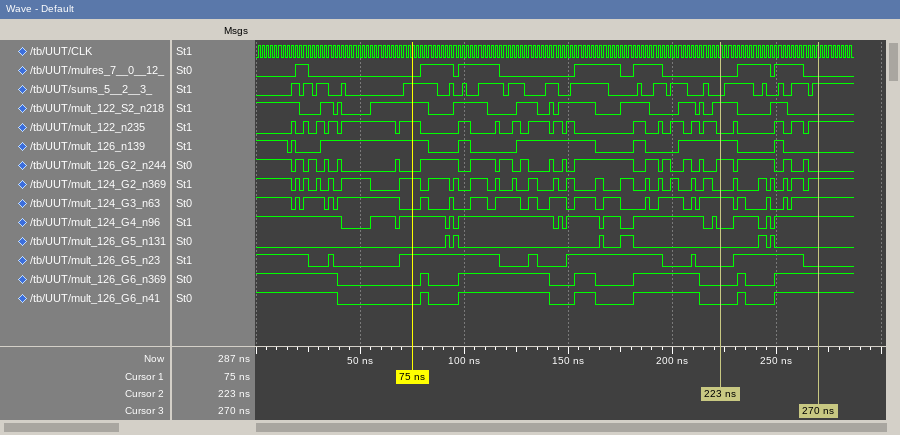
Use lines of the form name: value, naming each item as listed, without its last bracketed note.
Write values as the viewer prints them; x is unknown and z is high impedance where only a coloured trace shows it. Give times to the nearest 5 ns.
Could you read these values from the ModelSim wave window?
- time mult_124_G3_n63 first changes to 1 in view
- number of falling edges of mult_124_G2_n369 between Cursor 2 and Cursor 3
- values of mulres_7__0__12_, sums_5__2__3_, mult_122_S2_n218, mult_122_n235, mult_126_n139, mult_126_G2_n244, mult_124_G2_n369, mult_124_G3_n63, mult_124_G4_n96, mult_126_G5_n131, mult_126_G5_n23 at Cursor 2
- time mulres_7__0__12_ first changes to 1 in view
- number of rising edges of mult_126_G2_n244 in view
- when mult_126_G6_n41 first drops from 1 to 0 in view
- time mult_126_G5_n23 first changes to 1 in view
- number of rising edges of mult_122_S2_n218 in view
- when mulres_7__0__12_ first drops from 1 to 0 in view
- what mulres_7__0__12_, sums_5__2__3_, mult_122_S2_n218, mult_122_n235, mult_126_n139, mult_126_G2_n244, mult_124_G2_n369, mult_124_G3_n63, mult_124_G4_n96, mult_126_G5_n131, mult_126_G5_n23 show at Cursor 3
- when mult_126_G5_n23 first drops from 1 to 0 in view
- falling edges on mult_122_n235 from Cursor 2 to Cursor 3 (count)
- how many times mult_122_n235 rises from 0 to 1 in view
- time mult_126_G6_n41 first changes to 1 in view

time mult_124_G3_n63 first changes to 1 in view: 20 ns
number of falling edges of mult_124_G2_n369 between Cursor 2 and Cursor 3: 5
values of mulres_7__0__12_, sums_5__2__3_, mult_122_S2_n218, mult_122_n235, mult_126_n139, mult_126_G2_n244, mult_124_G2_n369, mult_124_G3_n63, mult_124_G4_n96, mult_126_G5_n131, mult_126_G5_n23 at Cursor 2: mulres_7__0__12_=0, sums_5__2__3_=0, mult_122_S2_n218=1, mult_122_n235=0, mult_126_n139=1, mult_126_G2_n244=1, mult_124_G2_n369=0, mult_124_G3_n63=1, mult_124_G4_n96=0, mult_126_G5_n131=0, mult_126_G5_n23=0
time mulres_7__0__12_ first changes to 1 in view: 20 ns
number of rising edges of mult_126_G2_n244 in view: 20
when mult_126_G6_n41 first drops from 1 to 0 in view: 40 ns
time mult_126_G5_n23 first changes to 1 in view: 35 ns
number of rising edges of mult_122_S2_n218 in view: 12
when mulres_7__0__12_ first drops from 1 to 0 in view: 25 ns
what mulres_7__0__12_, sums_5__2__3_, mult_122_S2_n218, mult_122_n235, mult_126_n139, mult_126_G2_n244, mult_124_G2_n369, mult_124_G3_n63, mult_124_G4_n96, mult_126_G5_n131, mult_126_G5_n23 show at Cursor 3: mulres_7__0__12_=0, sums_5__2__3_=1, mult_122_S2_n218=0, mult_122_n235=1, mult_126_n139=0, mult_126_G2_n244=0, mult_124_G2_n369=1, mult_124_G3_n63=1, mult_124_G4_n96=1, mult_126_G5_n131=0, mult_126_G5_n23=0
when mult_126_G5_n23 first drops from 1 to 0 in view: 25 ns
falling edges on mult_122_n235 from Cursor 2 to Cursor 3: 3
how many times mult_122_n235 rises from 0 to 1 in view: 21
time mult_126_G6_n41 first changes to 1 in view: 80 ns
